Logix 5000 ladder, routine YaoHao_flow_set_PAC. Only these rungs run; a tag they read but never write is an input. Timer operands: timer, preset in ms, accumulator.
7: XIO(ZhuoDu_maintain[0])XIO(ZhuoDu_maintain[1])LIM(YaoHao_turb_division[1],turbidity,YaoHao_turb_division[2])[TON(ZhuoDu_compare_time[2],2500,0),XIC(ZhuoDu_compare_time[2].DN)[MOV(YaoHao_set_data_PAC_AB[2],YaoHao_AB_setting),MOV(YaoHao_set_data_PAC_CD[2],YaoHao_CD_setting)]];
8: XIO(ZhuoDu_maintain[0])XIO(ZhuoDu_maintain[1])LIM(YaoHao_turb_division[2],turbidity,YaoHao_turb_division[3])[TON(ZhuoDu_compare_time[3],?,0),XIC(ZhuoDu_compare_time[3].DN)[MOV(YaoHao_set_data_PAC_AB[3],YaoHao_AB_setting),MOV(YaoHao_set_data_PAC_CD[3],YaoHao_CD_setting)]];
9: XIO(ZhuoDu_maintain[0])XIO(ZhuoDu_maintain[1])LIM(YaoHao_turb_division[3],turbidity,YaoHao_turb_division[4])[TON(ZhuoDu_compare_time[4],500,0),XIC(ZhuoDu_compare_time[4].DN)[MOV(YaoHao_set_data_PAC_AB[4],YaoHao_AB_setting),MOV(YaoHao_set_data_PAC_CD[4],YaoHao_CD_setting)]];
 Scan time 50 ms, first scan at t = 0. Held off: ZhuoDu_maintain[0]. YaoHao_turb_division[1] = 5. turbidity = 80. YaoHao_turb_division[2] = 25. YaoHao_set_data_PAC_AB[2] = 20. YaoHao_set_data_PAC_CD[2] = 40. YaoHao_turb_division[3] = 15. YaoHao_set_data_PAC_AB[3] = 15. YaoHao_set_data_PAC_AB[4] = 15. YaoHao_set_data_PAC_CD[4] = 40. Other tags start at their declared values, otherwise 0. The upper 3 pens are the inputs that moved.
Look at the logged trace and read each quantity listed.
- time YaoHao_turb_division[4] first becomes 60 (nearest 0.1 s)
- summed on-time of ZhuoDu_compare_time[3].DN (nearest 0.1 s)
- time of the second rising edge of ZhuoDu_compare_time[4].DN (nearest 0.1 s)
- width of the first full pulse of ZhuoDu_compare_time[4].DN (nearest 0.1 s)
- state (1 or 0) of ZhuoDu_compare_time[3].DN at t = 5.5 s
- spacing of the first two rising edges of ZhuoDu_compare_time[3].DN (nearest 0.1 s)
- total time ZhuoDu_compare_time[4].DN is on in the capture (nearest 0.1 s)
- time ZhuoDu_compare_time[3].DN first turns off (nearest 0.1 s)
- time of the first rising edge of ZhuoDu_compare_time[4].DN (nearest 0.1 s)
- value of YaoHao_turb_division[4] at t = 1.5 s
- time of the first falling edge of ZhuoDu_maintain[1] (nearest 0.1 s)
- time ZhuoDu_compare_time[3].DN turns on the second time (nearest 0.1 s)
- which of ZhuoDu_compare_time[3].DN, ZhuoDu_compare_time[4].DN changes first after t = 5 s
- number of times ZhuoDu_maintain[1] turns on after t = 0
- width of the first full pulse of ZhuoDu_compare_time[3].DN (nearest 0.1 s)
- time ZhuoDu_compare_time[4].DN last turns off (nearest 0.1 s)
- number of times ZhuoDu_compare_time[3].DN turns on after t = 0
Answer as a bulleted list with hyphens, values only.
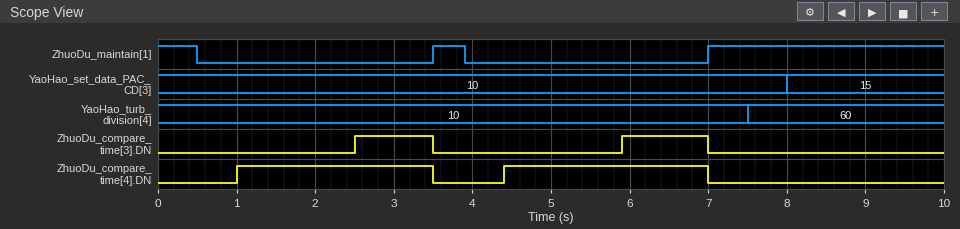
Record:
- 7.5 s
- 2.1 s
- 4.4 s
- 2.5 s
- 0
- 3.4 s
- 5.1 s
- 3.5 s
- 1.0 s
- 10
- 0.5 s
- 5.9 s
- ZhuoDu_compare_time[3].DN
- 2
- 1.0 s
- 7.0 s
- 2
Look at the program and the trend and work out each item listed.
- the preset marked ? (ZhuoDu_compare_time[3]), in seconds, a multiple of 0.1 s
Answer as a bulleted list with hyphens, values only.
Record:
- 2.0 s
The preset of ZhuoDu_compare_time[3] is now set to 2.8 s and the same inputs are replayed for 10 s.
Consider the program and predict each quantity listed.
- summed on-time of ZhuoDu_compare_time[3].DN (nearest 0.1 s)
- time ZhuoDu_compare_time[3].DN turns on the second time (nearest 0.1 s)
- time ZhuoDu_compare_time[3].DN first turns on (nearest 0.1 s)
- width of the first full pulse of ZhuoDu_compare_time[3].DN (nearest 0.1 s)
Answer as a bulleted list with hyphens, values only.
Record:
- 0.5 s
- 6.7 s
- 3.3 s
- 0.2 s
